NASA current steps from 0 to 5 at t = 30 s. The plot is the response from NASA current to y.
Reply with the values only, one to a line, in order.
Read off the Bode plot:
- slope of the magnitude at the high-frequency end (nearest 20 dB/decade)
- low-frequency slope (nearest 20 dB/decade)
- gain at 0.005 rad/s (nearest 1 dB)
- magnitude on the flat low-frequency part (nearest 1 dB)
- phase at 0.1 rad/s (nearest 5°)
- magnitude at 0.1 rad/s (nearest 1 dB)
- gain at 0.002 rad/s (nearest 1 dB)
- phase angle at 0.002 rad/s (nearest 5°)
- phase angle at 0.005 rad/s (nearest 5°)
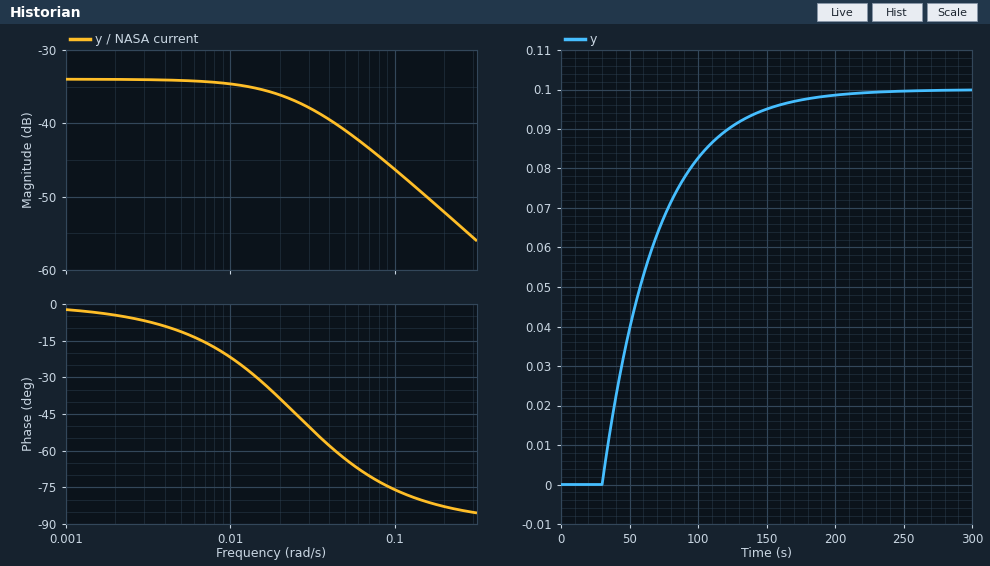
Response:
-20 dB/decade
0 dB/decade
-34 dB
-34 dB
-75°
-46 dB
-34 dB
-5°
-10°
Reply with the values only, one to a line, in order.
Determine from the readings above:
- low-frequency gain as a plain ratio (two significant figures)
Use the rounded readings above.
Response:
0.020
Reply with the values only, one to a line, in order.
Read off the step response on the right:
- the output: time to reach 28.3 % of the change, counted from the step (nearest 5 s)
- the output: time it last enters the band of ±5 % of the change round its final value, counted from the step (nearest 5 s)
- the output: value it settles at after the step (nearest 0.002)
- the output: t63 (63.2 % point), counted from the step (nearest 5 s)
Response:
15 s
120 s
0.100
40 s
